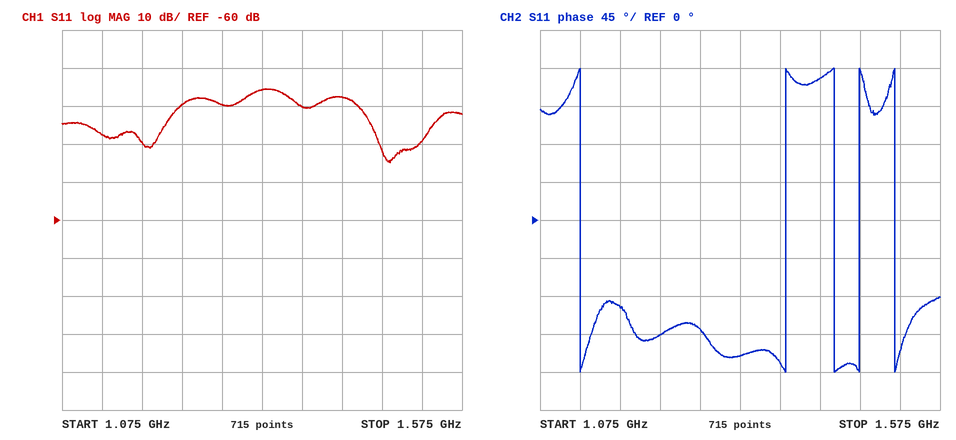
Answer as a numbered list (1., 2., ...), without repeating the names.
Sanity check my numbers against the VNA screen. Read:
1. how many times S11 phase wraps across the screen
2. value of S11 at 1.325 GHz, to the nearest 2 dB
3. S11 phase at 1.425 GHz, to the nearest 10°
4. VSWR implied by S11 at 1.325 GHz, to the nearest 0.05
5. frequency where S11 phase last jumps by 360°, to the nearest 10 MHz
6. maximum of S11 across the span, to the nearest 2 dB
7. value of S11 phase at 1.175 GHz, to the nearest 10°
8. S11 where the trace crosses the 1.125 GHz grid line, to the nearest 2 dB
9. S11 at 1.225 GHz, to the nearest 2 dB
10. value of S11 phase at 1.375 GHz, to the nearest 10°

1. 5
2. -26 dB
3. 170°
4. 1.10
5. 1.52 GHz
6. -26 dB
7. -100°
8. -38 dB
9. -30 dB
10. -170°
